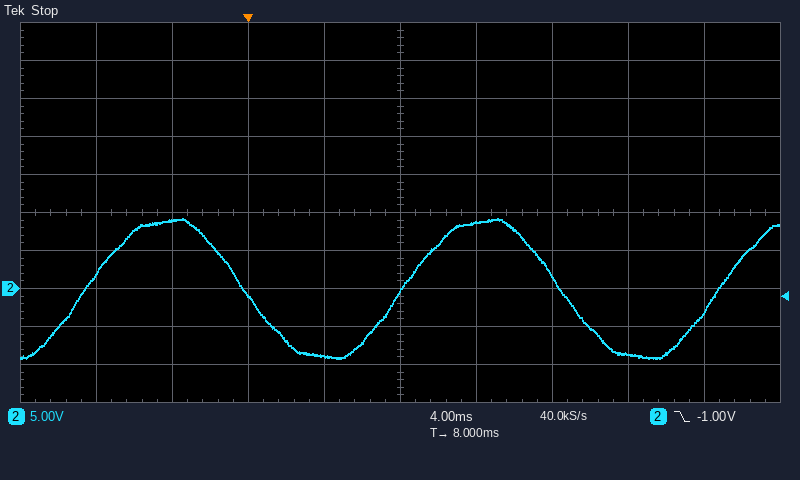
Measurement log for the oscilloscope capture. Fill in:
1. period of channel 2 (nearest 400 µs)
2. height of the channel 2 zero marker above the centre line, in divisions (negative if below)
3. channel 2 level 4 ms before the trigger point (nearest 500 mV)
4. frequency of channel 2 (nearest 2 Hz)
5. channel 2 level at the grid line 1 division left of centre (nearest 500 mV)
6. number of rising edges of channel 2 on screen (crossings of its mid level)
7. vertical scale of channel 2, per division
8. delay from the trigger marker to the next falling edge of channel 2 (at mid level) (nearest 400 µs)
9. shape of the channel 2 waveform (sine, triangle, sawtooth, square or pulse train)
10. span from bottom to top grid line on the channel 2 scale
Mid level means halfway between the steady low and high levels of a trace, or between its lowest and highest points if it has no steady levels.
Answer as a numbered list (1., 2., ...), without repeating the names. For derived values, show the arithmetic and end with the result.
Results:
1. 16.8 ms
2. -2.0 div
3. 9.0 V
4. 1 / 16.8 ms ≈ 60 Hz
5. -9.0 V
6. 3
7. 5 V
8. 16.4 ms
9. sine
10. 50 V
